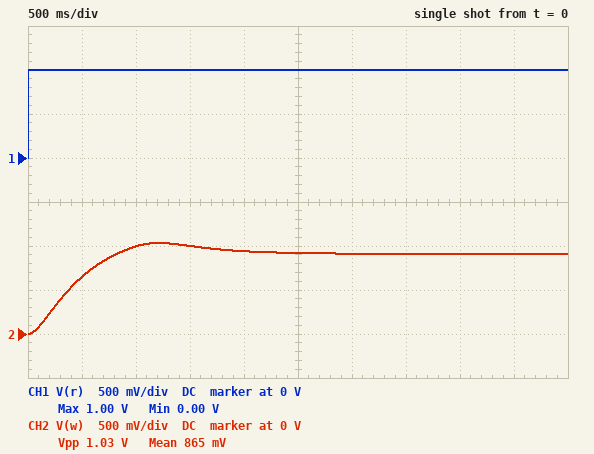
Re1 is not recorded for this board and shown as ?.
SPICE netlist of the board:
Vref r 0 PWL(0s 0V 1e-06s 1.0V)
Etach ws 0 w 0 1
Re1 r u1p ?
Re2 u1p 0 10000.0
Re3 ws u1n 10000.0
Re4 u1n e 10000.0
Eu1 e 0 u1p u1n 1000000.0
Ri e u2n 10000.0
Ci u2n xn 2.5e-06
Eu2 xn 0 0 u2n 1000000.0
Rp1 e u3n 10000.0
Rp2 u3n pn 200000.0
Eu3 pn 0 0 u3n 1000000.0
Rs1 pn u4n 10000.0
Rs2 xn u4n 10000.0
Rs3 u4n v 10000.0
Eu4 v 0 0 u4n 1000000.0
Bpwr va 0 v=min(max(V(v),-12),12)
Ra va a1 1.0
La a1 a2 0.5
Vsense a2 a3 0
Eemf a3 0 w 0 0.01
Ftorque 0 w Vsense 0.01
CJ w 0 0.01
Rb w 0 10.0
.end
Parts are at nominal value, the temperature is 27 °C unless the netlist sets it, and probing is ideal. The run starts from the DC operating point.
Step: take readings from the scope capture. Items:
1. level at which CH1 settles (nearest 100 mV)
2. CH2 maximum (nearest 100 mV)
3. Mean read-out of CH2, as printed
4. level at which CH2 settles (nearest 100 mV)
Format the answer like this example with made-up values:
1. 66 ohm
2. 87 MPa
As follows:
1. 1.0 V
2. 1.0 V
3. 865 mV
4. 900 mV
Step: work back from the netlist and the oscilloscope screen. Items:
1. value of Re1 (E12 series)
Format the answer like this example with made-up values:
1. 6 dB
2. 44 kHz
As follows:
1. 12 kΩ
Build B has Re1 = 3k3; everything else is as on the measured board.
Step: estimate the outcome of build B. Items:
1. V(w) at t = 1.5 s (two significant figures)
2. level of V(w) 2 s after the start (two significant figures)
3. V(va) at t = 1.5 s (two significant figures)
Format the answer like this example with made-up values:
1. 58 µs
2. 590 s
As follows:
1. 1.1 V
2. 1.2 V
3. 12 V
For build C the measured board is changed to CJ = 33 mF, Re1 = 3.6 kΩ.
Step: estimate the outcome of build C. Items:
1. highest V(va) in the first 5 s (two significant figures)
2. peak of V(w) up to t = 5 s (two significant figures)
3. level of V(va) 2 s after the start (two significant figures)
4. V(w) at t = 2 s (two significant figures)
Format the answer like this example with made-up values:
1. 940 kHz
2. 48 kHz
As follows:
1. 12 V
2. 1.2 V
3. 12 V
4. 1.1 V
